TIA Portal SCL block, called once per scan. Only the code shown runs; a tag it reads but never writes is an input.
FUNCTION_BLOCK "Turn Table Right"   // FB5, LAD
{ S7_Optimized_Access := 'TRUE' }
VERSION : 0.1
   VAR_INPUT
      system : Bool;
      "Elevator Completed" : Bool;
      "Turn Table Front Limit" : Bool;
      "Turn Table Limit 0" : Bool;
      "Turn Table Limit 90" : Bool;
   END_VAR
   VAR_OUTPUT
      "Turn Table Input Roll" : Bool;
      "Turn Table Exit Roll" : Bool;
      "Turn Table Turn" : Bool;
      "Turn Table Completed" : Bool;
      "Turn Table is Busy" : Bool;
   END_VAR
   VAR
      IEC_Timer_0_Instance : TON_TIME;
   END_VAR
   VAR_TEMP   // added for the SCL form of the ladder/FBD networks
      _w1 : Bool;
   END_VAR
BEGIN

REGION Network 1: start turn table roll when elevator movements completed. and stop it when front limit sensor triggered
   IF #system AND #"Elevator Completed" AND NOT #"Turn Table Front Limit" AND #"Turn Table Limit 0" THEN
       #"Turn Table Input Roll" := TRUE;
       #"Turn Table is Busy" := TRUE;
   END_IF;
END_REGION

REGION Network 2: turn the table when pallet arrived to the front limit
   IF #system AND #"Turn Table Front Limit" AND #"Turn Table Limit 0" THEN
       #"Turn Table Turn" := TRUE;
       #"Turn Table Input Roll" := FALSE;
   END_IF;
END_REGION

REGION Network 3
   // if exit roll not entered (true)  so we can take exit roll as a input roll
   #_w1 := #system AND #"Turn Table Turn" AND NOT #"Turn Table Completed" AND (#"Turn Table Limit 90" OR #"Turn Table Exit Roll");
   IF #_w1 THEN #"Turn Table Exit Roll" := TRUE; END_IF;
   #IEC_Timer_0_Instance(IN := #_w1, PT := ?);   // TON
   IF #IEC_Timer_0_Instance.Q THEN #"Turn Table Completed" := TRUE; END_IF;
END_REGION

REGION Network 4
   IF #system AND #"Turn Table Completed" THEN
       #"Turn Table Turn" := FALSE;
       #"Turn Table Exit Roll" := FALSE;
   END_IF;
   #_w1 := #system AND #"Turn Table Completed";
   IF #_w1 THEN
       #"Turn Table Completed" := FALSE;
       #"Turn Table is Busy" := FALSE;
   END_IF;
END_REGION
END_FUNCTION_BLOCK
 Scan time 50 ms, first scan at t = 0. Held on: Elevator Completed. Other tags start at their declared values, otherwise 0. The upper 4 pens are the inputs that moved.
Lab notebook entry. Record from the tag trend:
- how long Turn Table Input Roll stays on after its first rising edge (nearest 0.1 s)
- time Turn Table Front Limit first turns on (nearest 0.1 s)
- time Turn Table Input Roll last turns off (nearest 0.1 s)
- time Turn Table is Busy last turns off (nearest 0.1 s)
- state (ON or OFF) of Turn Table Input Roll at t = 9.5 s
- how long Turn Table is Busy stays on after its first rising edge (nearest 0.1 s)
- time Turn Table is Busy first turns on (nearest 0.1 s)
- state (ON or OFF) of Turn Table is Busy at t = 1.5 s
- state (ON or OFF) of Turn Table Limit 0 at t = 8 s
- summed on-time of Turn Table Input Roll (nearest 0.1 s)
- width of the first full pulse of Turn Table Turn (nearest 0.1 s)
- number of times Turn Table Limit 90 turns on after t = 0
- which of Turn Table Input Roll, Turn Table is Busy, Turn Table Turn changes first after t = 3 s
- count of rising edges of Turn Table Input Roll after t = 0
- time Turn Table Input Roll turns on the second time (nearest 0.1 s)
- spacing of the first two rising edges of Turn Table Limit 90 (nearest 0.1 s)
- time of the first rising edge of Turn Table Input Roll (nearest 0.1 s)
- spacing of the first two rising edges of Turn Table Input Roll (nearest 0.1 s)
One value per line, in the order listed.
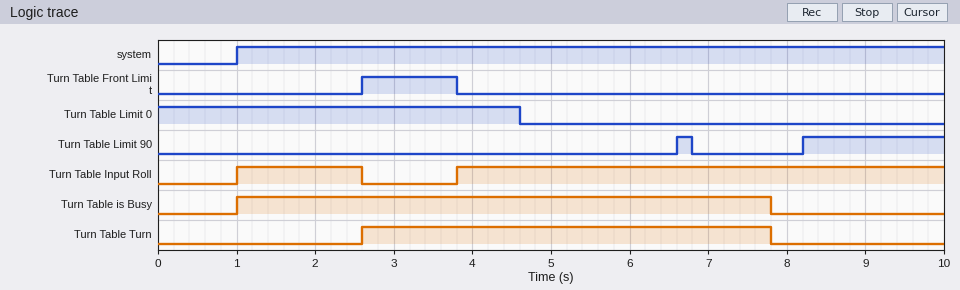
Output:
1.6 s
2.6 s
2.6 s
7.8 s
ON
6.8 s
1.0 s
ON
OFF
7.8 s
5.2 s
2
Turn Table Input Roll
2
3.8 s
1.6 s
1.0 s
2.8 s
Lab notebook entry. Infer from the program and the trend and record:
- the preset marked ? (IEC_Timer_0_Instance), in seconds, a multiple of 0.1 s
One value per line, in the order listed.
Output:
1.2 s
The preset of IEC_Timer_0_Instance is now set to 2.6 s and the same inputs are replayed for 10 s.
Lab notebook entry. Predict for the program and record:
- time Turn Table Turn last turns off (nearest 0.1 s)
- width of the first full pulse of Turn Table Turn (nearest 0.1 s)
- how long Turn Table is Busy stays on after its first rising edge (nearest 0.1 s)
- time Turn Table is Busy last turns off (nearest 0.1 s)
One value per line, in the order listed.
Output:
9.2 s
6.6 s
8.2 s
9.2 s
